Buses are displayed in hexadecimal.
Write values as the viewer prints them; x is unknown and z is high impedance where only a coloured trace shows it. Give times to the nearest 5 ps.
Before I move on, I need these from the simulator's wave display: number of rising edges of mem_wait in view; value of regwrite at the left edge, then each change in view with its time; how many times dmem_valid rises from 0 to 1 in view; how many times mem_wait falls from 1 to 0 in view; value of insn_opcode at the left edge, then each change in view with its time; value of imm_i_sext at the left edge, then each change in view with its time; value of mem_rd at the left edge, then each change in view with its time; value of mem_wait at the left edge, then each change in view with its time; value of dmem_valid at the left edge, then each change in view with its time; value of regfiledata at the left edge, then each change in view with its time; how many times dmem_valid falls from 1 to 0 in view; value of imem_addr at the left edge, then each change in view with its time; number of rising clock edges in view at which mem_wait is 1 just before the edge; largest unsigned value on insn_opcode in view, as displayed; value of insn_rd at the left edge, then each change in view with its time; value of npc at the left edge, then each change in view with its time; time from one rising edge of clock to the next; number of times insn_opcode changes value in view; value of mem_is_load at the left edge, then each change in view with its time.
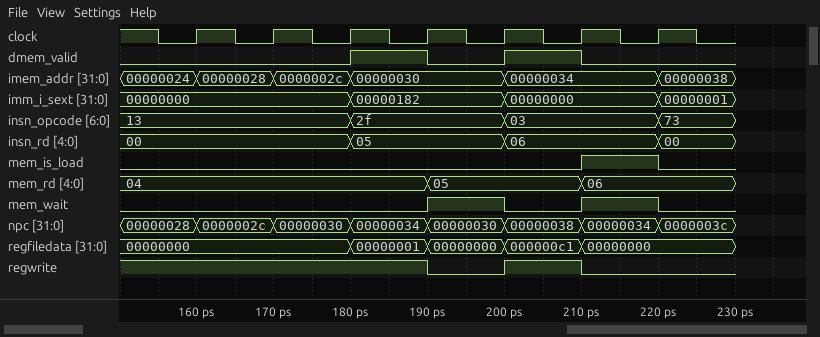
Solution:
2
1, 0 at 190 ps, 1 at 200 ps, 0 at 210 ps
2
2
13, 2f at 180 ps, 03 at 200 ps, 73 at 220 ps
00000000, 00000182 at 180 ps, 00000000 at 200 ps, 00000001 at 220 ps
04, 05 at 190 ps, 06 at 210 ps
0, 1 at 190 ps, 0 at 200 ps, 1 at 210 ps, 0 at 220 ps
0, 1 at 180 ps, 0 at 190 ps, 1 at 200 ps, 0 at 210 ps
00000000, 00000001 at 180 ps, 00000000 at 190 ps, 000000c1 at 200 ps, 00000000 at 210 ps
2
00000024, 00000028 at 160 ps, 0000002c at 170 ps, 00000030 at 180 ps, 00000034 at 200 ps, 00000038 at 220 ps
2
73
00, 05 at 180 ps, 06 at 200 ps, 00 at 220 ps
00000028, 0000002c at 160 ps, 00000030 at 170 ps, 00000034 at 180 ps, 00000030 at 190 ps, 00000038 at 200 ps, 00000034 at 210 ps, 0000003c at 220 ps
10 ps
3
0, 1 at 210 ps, 0 at 220 ps
